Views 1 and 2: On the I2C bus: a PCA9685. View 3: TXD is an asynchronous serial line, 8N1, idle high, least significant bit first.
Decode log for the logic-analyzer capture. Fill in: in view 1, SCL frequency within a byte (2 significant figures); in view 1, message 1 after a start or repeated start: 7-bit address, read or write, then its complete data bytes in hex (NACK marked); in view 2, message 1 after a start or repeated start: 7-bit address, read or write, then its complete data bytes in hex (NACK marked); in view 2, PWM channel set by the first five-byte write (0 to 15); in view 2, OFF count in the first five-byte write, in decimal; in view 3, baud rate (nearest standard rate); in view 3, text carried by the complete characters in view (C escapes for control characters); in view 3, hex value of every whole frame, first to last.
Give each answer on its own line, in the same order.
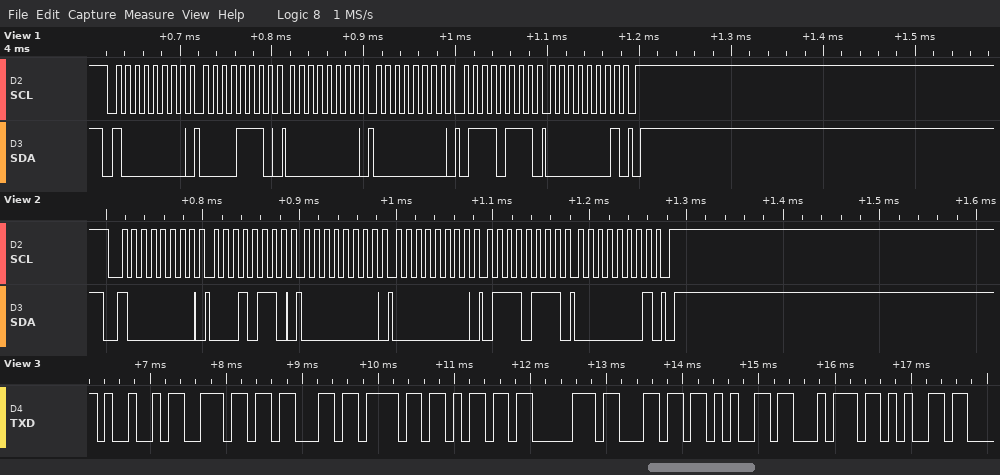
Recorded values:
100 kHz
0x40 write: 0E 00 00 77 01
0x40 write: 16 00 00 77 01
4
375
9600 baud
"Incomplete"
49 6E 63 6F 6D 70 6C 65 74 65
